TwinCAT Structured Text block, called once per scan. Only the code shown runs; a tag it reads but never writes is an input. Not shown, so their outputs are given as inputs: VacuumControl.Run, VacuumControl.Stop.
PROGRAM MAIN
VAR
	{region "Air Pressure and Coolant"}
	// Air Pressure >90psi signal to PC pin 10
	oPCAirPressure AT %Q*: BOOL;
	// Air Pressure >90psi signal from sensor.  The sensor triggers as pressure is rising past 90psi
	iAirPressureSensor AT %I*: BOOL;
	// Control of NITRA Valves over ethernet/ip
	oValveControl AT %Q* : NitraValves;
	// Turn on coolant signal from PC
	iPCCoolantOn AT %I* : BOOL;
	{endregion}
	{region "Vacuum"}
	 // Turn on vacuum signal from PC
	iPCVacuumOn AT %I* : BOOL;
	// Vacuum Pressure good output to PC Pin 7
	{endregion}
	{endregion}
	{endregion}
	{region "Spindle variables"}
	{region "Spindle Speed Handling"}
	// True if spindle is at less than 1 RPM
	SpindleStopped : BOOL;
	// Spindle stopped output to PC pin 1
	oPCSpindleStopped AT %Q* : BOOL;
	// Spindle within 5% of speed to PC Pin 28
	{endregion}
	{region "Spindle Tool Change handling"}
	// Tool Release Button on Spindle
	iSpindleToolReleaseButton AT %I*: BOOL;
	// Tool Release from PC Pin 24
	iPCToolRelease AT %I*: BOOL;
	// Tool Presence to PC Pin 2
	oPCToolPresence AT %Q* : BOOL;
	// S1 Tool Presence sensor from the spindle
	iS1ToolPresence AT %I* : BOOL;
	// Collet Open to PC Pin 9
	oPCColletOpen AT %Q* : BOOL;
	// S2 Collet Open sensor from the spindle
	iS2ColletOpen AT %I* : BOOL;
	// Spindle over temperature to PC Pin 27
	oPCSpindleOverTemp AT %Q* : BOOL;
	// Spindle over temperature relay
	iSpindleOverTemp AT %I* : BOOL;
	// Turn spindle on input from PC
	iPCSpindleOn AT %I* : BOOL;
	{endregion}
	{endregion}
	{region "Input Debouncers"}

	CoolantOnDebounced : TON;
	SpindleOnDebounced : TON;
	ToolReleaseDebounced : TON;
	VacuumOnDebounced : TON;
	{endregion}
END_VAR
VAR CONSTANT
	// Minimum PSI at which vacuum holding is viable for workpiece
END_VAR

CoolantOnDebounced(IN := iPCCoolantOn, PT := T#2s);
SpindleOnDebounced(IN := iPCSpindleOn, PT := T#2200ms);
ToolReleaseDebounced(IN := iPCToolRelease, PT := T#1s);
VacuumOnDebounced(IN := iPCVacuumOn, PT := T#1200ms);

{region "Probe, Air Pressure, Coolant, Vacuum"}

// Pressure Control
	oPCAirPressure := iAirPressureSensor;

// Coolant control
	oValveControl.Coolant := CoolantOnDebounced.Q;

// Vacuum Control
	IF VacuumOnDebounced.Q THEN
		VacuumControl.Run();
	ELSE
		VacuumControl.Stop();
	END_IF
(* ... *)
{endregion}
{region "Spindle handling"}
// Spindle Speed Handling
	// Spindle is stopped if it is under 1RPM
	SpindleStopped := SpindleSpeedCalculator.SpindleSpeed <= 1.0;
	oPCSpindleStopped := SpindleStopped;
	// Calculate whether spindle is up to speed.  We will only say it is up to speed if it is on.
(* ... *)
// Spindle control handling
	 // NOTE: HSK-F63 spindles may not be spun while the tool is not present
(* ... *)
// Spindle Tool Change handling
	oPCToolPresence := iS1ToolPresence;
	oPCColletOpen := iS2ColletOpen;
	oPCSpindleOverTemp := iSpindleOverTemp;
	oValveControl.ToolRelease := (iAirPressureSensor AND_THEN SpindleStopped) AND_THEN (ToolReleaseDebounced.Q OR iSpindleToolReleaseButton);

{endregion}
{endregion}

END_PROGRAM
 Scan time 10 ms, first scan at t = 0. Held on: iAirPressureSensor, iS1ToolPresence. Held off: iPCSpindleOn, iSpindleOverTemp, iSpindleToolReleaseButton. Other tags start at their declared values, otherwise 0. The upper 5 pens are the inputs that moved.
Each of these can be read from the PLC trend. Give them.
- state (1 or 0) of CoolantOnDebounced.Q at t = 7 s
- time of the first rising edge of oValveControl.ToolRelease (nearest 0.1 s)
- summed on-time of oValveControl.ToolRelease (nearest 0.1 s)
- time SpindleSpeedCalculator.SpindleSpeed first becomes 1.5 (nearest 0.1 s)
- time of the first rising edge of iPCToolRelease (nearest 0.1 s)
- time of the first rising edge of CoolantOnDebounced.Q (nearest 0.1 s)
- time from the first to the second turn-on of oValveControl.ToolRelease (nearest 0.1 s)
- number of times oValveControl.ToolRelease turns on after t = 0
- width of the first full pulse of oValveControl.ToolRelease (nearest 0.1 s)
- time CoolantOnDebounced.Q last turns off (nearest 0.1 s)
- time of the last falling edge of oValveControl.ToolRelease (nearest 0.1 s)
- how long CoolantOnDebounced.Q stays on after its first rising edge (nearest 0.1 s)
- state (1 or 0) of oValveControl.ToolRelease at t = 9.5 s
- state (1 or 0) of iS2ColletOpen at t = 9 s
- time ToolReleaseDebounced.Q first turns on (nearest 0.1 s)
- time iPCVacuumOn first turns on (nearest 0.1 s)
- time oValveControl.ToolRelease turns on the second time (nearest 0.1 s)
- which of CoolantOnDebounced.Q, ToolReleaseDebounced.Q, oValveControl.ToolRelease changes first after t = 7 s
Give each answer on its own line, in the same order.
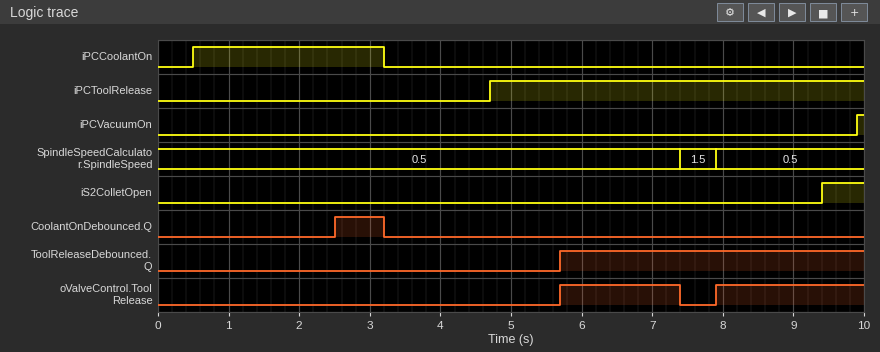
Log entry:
0
5.7 s
3.8 s
7.4 s
4.7 s
2.5 s
2.2 s
2
1.7 s
3.2 s
7.4 s
0.7 s
1
0
5.7 s
9.9 s
7.9 s
oValveControl.ToolRelease
